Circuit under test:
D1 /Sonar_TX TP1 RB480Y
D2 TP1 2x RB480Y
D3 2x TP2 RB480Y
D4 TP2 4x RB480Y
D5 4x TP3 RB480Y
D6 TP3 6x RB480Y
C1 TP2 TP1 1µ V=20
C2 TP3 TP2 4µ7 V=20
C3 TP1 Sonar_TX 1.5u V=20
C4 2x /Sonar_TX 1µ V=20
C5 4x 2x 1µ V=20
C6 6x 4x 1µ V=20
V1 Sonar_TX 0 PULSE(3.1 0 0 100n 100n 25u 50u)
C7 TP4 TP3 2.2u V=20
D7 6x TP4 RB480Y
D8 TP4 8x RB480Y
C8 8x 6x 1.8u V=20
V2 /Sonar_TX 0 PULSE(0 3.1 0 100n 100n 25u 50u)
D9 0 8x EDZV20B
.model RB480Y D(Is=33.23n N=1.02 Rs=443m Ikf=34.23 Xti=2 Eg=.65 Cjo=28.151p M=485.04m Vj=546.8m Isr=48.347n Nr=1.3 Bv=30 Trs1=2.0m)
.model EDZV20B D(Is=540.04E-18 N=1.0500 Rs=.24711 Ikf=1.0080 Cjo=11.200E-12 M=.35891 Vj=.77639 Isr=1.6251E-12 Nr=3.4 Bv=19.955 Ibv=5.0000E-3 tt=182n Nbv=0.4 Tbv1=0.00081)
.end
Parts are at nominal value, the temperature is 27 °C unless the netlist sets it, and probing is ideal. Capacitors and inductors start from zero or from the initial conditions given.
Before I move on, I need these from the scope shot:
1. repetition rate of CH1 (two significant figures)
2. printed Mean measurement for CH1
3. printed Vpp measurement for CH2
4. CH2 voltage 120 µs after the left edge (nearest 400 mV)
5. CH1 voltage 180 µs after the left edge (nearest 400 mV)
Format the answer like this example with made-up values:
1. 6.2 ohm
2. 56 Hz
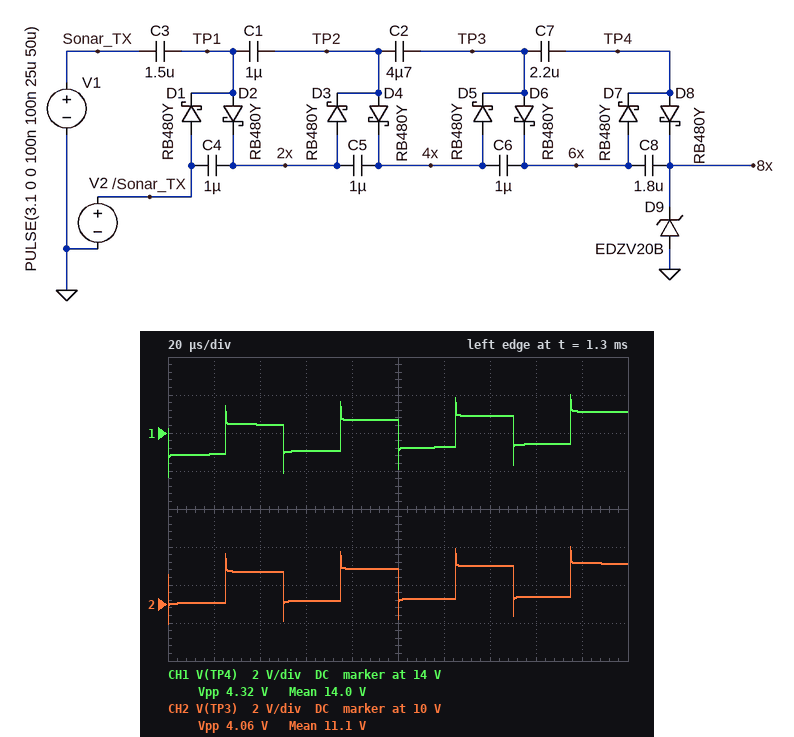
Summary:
1. 20 kHz
2. 14.0 V
3. 4.06 V
4. 10.4 V
5. 15.2 V
